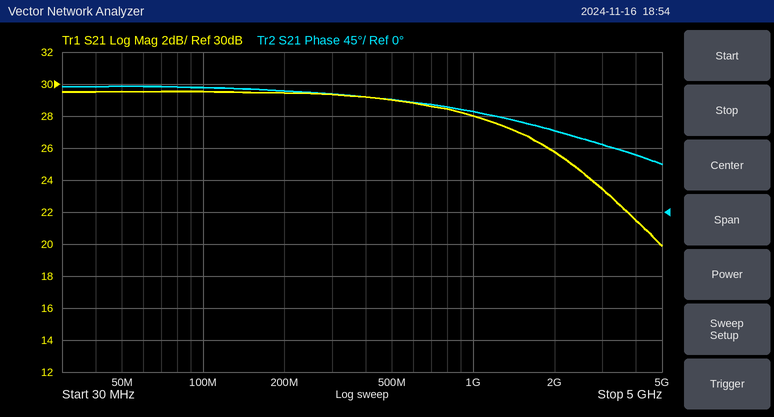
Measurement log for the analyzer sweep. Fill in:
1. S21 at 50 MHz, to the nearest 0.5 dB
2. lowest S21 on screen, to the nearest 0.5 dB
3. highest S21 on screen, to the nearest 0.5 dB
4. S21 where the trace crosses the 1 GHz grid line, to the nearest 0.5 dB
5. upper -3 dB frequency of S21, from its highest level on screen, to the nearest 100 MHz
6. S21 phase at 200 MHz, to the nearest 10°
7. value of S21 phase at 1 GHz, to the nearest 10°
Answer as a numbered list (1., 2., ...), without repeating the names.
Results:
1. 29.5 dB
2. 20.0 dB
3. 29.5 dB
4. 28.0 dB
5. 1.7 GHz
6. 170°
7. 140°
